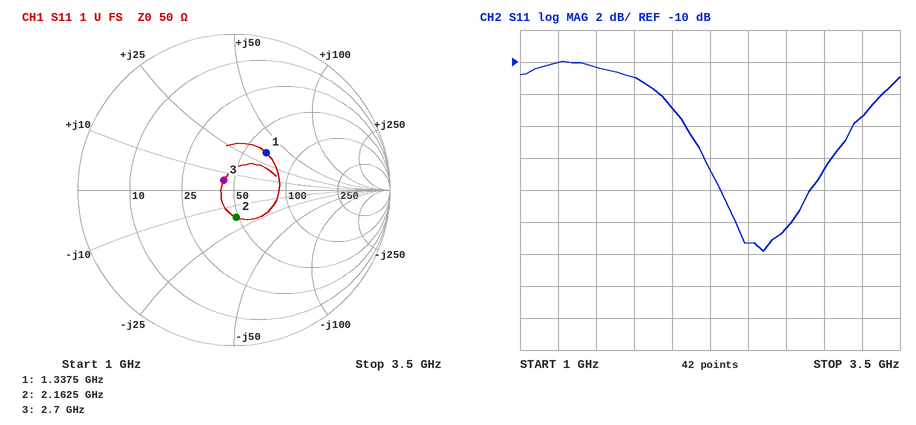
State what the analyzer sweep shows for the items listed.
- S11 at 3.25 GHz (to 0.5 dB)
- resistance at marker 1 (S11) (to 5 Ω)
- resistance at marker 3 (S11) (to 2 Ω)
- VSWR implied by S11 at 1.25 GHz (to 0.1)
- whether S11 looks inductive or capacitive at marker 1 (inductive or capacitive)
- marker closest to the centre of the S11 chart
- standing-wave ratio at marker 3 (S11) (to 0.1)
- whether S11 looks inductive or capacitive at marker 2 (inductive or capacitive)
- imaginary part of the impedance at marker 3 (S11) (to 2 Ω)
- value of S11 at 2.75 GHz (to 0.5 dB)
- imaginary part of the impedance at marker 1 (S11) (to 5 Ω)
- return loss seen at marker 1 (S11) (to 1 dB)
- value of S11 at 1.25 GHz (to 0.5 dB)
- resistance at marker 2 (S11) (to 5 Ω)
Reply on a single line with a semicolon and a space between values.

-13.5 dB; 65 Ω; 44 Ω; 1.9; inductive; marker 3; 1.2; capacitive; +6 Ω; -20.5 dB; +35 Ω; 10 dB; -10.0 dB; 50 Ω
